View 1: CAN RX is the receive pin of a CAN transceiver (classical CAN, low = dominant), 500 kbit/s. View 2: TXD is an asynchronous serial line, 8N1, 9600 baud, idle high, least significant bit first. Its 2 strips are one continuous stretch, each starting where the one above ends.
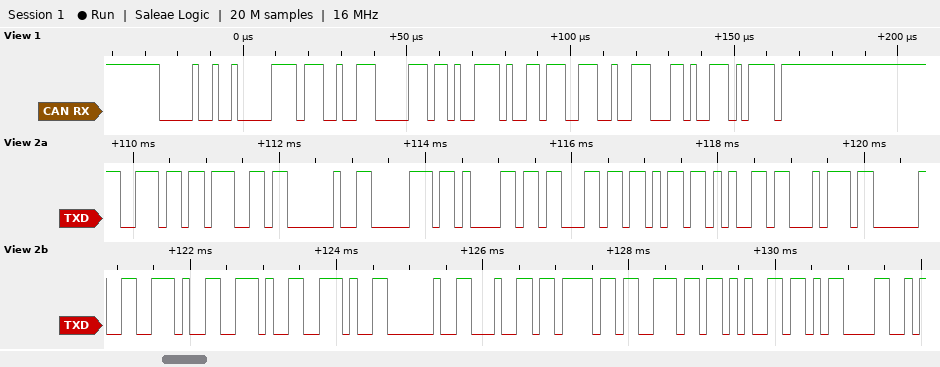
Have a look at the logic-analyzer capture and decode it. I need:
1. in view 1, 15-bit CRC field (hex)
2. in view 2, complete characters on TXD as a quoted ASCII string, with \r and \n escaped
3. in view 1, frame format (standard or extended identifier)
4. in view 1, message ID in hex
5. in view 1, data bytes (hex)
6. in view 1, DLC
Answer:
0x69D7
"ng packet ... done\r"
standard
0x012
72 70 6D 3D 37 39 38
7
